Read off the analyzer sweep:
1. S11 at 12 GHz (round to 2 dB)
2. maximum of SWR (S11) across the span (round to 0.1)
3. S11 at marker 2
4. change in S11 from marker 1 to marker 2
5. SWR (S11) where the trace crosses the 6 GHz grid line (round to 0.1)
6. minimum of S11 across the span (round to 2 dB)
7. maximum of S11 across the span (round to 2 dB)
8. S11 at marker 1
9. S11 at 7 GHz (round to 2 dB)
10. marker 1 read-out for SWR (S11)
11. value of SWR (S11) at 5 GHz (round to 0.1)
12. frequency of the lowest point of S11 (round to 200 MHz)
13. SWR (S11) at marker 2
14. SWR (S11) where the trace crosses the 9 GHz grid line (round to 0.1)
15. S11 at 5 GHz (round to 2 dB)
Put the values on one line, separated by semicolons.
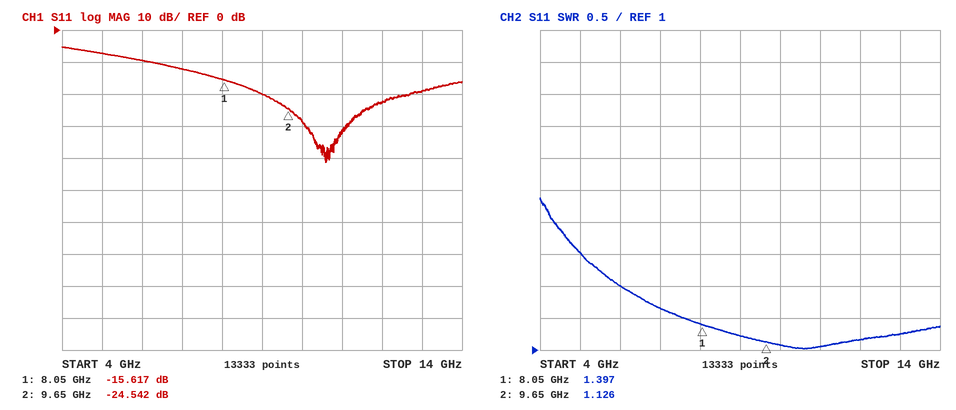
-22 dB; 3.4; -24.542 dB; -8.925 dB; 2.0; -42 dB; -6 dB; -15.617 dB; -12 dB; 1.397; 2.5; 10.6 GHz; 1.126; 1.2; -8 dB
